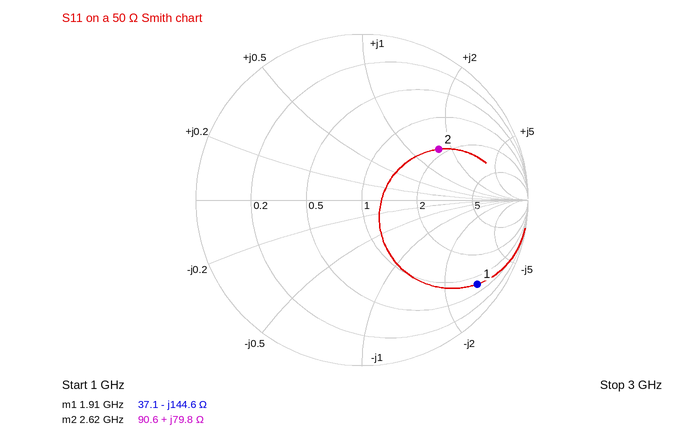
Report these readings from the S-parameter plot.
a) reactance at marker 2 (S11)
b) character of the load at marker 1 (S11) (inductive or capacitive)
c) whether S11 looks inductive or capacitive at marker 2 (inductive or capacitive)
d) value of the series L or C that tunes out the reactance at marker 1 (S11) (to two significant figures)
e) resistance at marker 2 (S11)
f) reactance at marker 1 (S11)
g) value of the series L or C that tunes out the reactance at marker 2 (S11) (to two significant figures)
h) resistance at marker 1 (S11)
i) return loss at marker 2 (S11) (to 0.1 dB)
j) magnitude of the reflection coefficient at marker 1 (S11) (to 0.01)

+79.8 Ω
capacitive
inductive
12 nH
90.6 Ω
-144.6 Ω
760 fF
37.1 Ω
5.1 dB
0.86
